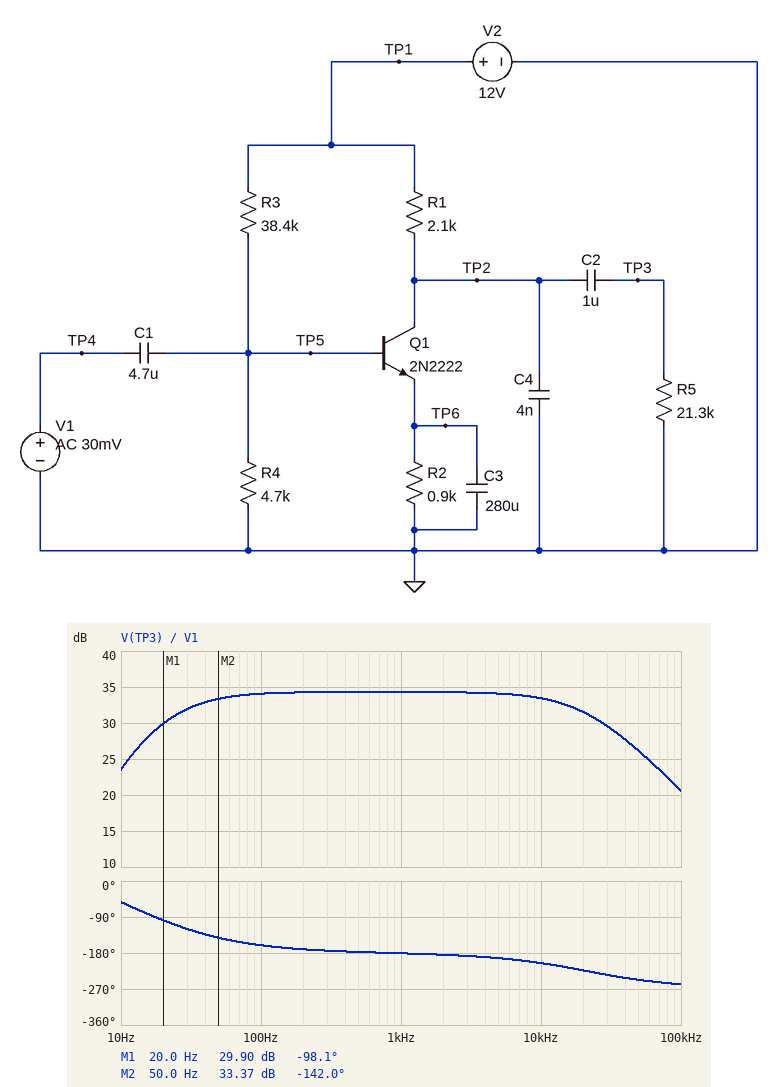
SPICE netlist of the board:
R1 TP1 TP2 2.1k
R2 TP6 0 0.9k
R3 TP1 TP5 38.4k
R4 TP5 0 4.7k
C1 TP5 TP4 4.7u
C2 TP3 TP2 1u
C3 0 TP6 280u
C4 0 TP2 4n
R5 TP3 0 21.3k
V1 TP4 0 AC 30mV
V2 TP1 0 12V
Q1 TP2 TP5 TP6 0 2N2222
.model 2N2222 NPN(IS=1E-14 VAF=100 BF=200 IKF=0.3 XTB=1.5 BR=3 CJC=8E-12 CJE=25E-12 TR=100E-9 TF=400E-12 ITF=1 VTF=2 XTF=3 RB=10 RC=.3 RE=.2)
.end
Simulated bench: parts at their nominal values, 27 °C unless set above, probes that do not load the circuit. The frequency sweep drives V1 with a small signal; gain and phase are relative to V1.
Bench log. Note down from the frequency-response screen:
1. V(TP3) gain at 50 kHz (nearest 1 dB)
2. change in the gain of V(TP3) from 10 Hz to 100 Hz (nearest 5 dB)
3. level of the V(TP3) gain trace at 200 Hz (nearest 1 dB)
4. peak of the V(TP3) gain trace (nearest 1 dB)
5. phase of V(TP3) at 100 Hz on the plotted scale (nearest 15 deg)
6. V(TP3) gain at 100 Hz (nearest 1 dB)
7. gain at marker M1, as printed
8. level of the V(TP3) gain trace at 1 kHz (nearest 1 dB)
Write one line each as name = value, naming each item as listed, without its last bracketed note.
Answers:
V(TP3) gain at 50 kHz = 26 dB
change in the gain of V(TP3) from 10 Hz to 100 Hz = 10 dB
level of the V(TP3) gain trace at 200 Hz = 34 dB
peak of the V(TP3) gain trace = 34 dB
phase of V(TP3) at 100 Hz on the plotted scale = -165 deg
V(TP3) gain at 100 Hz = 34 dB
gain at marker M1, as printed = 29.90 dB
level of the V(TP3) gain trace at 1 kHz = 34 dB
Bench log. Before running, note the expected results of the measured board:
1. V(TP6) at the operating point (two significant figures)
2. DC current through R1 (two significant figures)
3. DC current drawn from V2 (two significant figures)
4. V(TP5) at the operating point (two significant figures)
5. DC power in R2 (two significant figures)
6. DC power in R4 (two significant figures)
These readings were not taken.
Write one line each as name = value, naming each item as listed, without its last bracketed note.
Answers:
V(TP6) at the operating point = 650 mV
DC current through R1 = 720 µA
DC current drawn from V2 = 1.0 mA
V(TP5) at the operating point = 1.3 V
DC power in R2 = 470 µW
DC power in R4 = 360 µW
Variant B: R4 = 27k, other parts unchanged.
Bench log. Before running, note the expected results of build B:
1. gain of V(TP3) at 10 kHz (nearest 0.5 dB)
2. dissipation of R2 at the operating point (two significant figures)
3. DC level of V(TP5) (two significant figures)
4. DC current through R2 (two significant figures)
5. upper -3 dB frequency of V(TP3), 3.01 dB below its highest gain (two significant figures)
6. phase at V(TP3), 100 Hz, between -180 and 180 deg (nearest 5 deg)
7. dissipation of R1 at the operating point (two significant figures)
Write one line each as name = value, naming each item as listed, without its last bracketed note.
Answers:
gain of V(TP3) at 10 kHz = 29.0 dB
dissipation of R2 at the operating point = 14 mW
DC level of V(TP5) = 4.3 V
DC current through R2 = 4.0 mA
upper -3 dB frequency of V(TP3), 3.01 dB below its highest gain = 170 kHz
phase at V(TP3), 100 Hz, between -180 and 180 deg = -90 deg
dissipation of R1 at the operating point = 33 mW
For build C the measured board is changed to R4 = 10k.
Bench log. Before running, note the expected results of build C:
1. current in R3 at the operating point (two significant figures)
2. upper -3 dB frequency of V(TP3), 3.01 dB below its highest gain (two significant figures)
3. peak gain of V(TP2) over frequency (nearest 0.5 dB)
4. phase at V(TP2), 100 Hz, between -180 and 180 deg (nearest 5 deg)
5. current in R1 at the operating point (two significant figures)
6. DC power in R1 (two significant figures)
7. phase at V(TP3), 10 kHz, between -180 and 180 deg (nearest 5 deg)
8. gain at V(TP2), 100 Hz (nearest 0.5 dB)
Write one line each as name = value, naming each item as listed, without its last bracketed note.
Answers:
current in R3 at the operating point = 250 µA
upper -3 dB frequency of V(TP3), 3.01 dB below its highest gain = 22 kHz
peak gain of V(TP2) over frequency = 42.5 dB
phase at V(TP2), 100 Hz, between -180 and 180 deg = -150 deg
current in R1 at the operating point = 1.9 mA
DC power in R1 = 7.7 mW
phase at V(TP3), 10 kHz, between -180 and 180 deg = 155 deg
gain at V(TP2), 100 Hz = 41.5 dB
